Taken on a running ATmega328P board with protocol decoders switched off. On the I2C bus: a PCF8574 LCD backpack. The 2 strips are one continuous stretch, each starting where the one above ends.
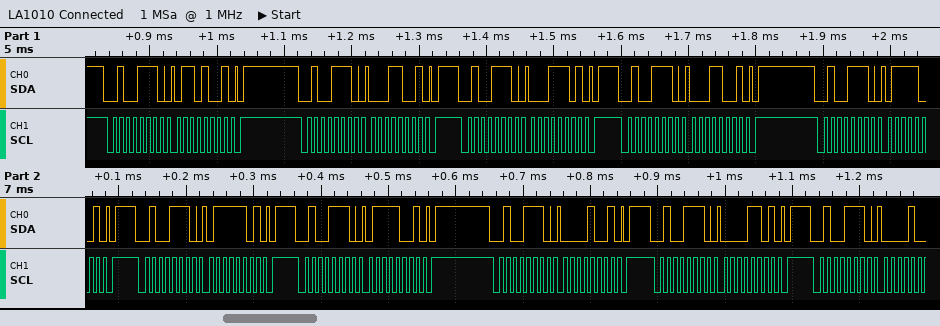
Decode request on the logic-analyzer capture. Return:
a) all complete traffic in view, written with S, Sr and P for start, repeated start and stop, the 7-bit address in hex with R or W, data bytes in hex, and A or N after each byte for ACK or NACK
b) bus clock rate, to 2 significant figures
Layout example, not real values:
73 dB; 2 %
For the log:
S 27W A 69 A P S 27W A 19 A P S 27W A 1D A P S 27W A 19 A P S 27W A 79 A P S 27W A 7D A P S 27W A 79 A P S 27W A 09 A P S 27W A 0D A P S 27W A; 100 kHz
